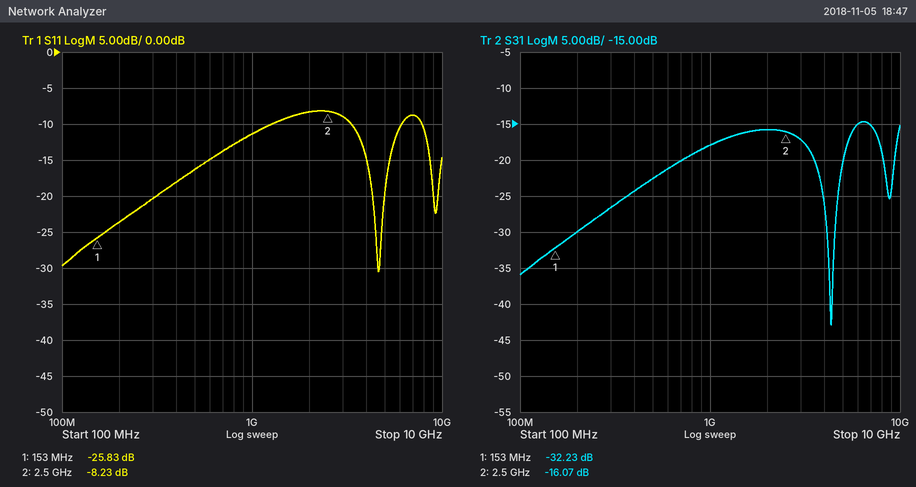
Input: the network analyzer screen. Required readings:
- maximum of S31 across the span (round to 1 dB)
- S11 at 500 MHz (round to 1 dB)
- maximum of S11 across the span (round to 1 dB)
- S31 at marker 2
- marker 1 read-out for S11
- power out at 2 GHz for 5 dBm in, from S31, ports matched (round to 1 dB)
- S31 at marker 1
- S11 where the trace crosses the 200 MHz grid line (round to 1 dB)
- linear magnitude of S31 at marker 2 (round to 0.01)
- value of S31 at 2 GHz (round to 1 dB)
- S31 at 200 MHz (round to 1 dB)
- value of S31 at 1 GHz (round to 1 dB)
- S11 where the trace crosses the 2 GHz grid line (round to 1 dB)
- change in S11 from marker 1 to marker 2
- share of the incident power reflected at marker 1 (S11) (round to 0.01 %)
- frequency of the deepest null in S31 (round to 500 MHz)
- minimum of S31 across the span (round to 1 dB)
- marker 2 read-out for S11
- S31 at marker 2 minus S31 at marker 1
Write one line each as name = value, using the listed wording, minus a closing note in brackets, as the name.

maximum of S31 across the span = -15 dB
S11 at 500 MHz = -16 dB
maximum of S11 across the span = -8 dB
S31 at marker 2 = -16.07 dB
marker 1 read-out for S11 = -25.83 dB
power out at 2 GHz for 5 dBm in, from S31, ports matched = -11 dBm
S31 at marker 1 = -32.23 dB
S11 where the trace crosses the 200 MHz grid line = -24 dB
linear magnitude of S31 at marker 2 = 0.16
value of S31 at 2 GHz = -16 dB
S31 at 200 MHz = -30 dB
value of S31 at 1 GHz = -18 dB
S11 where the trace crosses the 2 GHz grid line = -8 dB
change in S11 from marker 1 to marker 2 = 17.60 dB
share of the incident power reflected at marker 1 (S11) = 0.26 %
frequency of the deepest null in S31 = 4.5 GHz
minimum of S31 across the span = -43 dB
marker 2 read-out for S11 = -8.23 dB
S31 at marker 2 minus S31 at marker 1 = 16.16 dB
